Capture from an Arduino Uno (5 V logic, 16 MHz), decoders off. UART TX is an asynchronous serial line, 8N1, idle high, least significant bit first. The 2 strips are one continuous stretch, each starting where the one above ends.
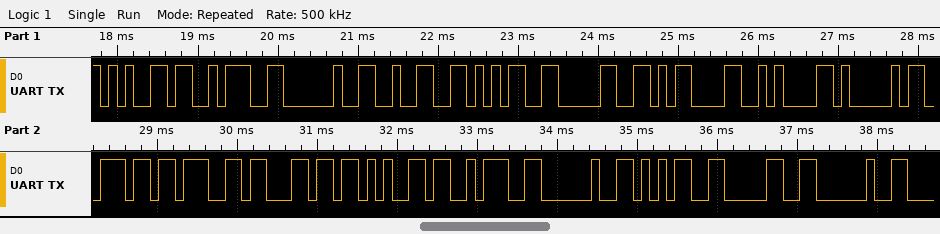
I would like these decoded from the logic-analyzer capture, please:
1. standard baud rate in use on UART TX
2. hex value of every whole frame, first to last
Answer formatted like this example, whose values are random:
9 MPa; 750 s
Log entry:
9600 baud; 0x65 0x3A 0x20 0x32 0x35 0x30 0x0D 0x0A 0x41 0x6E 0x67 0x6C 0x65 0x3A 0x20 0x35 0x30 0x20
